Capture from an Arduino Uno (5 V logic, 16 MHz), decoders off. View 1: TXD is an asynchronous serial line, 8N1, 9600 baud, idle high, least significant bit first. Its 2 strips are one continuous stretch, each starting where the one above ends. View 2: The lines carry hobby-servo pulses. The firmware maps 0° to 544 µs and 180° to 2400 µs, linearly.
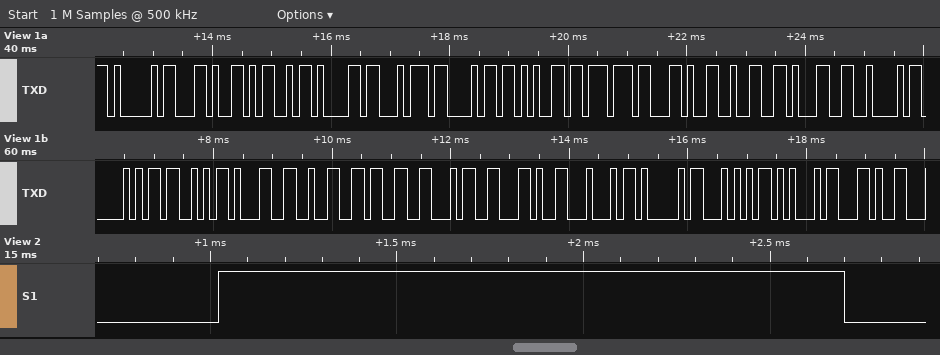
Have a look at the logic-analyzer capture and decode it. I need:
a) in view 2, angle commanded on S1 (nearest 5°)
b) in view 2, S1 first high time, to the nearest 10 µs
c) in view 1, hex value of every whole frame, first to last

110°
1680 µs
0x41 0x2C 0x4D 0x61 0x74 0x68 0x65 0x77 0x2C 0x32 0x31 0x42 0x50 0x53 0x31 0x32 0x33 0x34 0x2C 0x44 0x41 0x54 0x45 0x2C
